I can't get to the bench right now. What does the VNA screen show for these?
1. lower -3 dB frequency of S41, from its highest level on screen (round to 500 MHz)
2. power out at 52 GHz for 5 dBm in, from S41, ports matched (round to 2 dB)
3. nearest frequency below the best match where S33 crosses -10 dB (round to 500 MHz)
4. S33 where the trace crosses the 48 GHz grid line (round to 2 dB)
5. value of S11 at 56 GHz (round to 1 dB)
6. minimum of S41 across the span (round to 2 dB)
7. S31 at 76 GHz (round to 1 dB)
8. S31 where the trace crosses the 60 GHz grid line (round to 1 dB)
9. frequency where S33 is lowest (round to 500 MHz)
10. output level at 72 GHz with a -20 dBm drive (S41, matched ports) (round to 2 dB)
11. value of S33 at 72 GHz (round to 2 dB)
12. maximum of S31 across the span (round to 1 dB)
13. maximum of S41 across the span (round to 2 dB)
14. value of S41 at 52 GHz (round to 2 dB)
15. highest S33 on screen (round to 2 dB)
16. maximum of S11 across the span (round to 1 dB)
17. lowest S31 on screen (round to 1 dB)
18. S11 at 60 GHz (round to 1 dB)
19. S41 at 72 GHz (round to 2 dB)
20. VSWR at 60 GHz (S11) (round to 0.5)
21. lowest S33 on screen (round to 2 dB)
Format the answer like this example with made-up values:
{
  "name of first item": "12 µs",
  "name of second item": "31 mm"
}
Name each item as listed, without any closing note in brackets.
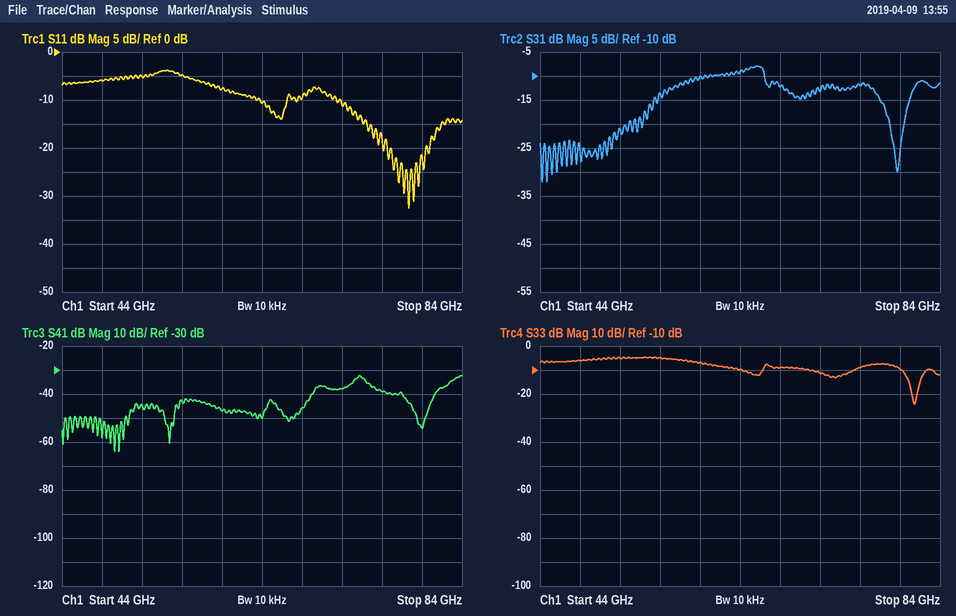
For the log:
{
  "lower -3 dB frequency of S41, from its highest level on screen": "73.0 GHz",
  "power out at 52 GHz for 5 dBm in, from S41, ports matched": "-40 dBm",
  "nearest frequency below the best match where S33 crosses -10 dB": "80.0 GHz",
  "S33 where the trace crosses the 48 GHz grid line": "-6 dB",
  "value of S11 at 56 GHz": "-5 dB",
  "minimum of S41 across the span": "-64 dB",
  "S31 at 76 GHz": "-12 dB",
  "S31 where the trace crosses the 60 GHz grid line": "-10 dB",
  "frequency where S33 is lowest": "81.5 GHz",
  "output level at 72 GHz with a -20 dBm drive (S41, matched ports)": "-58 dBm",
  "value of S33 at 72 GHz": "-12 dB",
  "maximum of S31 across the span": "-8 dB",
  "maximum of S41 across the span": "-32 dB",
  "value of S41 at 52 GHz": "-44 dB",
  "highest S33 on screen": "-4 dB",
  "maximum of S11 across the span": "-4 dB",
  "lowest S31 on screen": "-32 dB",
  "S11 at 60 GHz": "-8 dB",
  "S41 at 72 GHz": "-38 dB",
  "VSWR at 60 GHz (S11)": "2.5",
  "lowest S33 on screen": "-24 dB"
}
